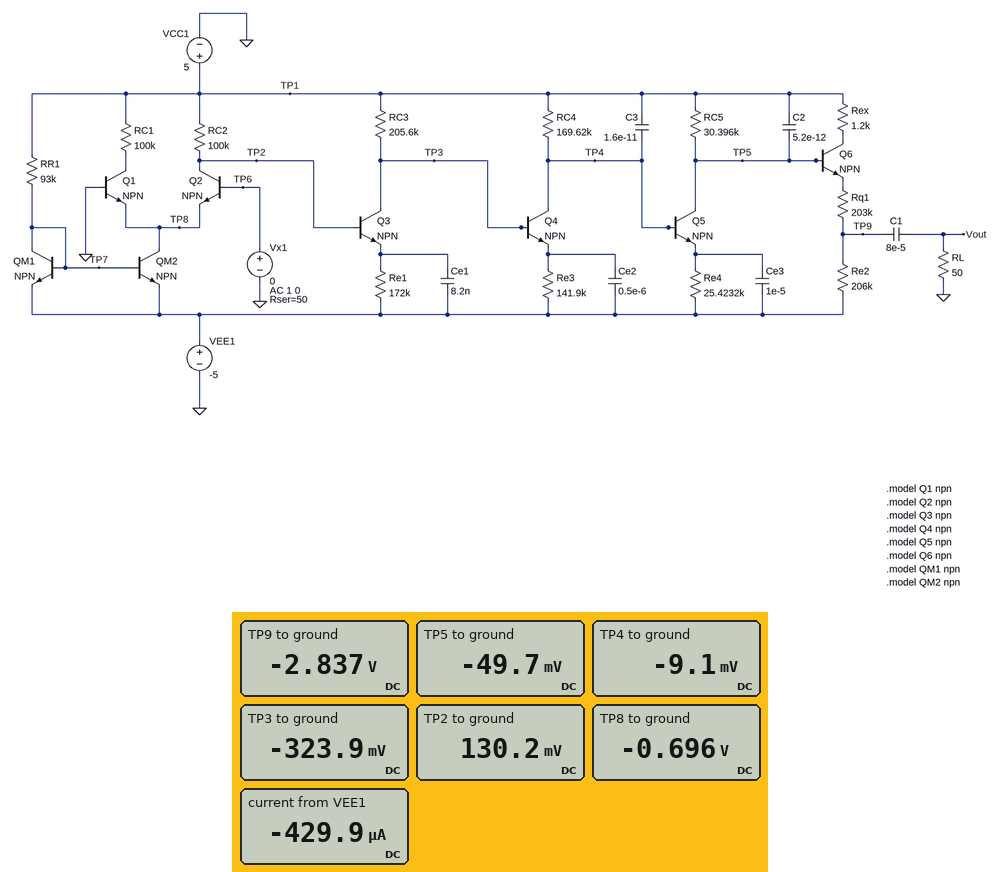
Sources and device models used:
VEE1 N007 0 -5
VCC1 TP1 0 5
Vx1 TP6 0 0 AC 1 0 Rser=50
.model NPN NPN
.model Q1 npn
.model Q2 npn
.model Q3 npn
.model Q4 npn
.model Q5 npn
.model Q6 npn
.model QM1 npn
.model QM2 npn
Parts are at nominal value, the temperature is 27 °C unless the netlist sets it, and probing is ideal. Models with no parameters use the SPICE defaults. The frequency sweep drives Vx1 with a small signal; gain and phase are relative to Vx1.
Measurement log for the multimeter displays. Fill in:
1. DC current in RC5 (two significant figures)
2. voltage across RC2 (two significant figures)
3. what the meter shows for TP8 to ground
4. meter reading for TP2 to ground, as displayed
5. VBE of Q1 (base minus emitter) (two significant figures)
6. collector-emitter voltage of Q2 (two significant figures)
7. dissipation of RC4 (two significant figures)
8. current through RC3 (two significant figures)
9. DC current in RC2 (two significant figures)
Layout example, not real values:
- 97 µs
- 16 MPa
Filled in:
- 170 µA
- 4.9 V
- -0.696 V
- 130.2 mV
- 700 mV
- 830 mV
- 150 µW
- 26 µA
- 49 µA
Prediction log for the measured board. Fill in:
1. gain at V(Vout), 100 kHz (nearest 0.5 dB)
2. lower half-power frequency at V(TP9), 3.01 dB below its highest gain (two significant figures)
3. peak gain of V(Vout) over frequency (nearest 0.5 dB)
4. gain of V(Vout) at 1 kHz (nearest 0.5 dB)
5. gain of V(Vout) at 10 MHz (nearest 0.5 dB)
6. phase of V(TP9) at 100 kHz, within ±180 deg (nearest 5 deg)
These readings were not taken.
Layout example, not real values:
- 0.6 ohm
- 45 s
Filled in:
- 63.0 dB
- 6.5 kHz
- 63.0 dB
- 46.5 dB
- 20.0 dB
- -10 deg
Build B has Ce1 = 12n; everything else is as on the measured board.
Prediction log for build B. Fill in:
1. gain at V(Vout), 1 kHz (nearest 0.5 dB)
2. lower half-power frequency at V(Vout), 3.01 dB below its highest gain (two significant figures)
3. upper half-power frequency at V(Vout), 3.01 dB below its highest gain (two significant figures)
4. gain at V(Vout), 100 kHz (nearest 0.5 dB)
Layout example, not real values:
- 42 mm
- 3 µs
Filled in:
- 49.5 dB
- 4.5 kHz
- 530 kHz
- 63.0 dB
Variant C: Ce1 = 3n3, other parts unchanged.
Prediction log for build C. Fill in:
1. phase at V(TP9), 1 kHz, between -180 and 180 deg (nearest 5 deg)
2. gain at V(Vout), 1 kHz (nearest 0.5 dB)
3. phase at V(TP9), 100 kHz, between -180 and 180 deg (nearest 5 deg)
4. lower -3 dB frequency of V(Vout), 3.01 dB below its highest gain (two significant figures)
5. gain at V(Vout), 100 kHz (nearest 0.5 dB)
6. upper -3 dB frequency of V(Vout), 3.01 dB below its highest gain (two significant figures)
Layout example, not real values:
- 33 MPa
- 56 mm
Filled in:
- 75 deg
- 39.0 dB
- -5 deg
- 16 kHz
- 62.5 dB
- 550 kHz
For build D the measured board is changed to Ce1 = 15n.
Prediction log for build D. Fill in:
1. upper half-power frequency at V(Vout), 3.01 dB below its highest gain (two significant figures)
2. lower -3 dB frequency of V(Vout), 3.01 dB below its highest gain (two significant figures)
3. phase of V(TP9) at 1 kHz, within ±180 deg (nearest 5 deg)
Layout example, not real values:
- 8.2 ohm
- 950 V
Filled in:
- 530 kHz
- 3.6 kHz
- 75 deg
